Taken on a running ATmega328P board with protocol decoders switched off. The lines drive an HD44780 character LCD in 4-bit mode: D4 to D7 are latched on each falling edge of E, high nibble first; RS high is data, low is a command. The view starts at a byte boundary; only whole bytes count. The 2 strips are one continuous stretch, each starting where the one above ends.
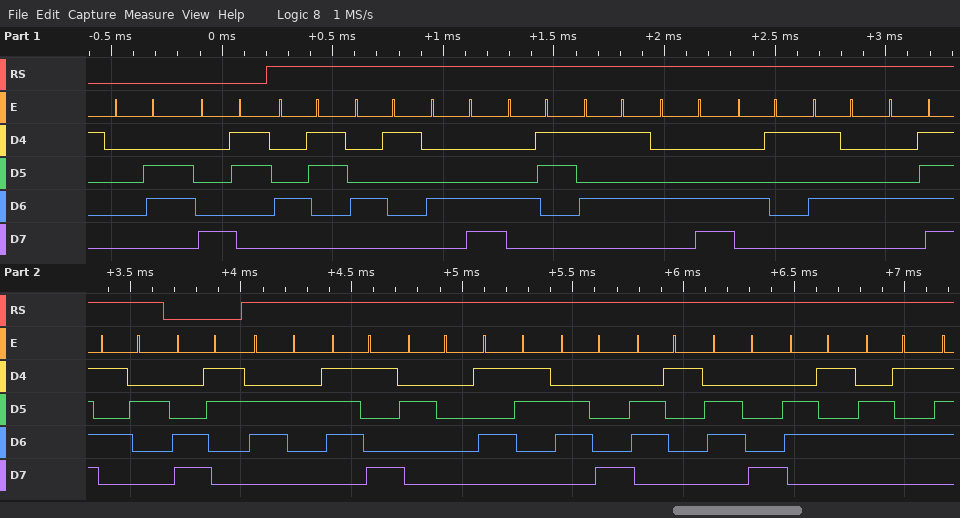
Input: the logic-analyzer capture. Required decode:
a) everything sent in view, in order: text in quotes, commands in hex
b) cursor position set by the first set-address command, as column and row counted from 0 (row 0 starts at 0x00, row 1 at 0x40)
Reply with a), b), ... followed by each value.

a) 0x06 0x83 "CALCULATOR" 0xC3 "by Shahee"
b) column 3, row 0
